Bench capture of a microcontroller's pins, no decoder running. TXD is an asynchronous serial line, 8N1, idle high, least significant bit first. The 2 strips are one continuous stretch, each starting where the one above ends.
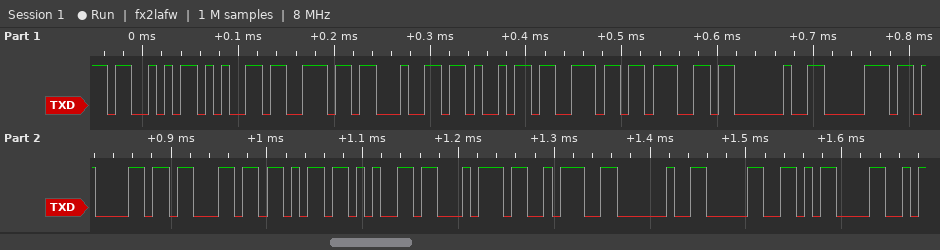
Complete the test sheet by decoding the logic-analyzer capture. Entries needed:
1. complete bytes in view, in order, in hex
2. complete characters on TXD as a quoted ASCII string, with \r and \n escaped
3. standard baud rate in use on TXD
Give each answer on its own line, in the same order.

53 65 6E 64 69 6E 67 20 70 61 63 6B 65 74 3A 20 30 0D
"Sending packet: 0\r"
115200 baud
